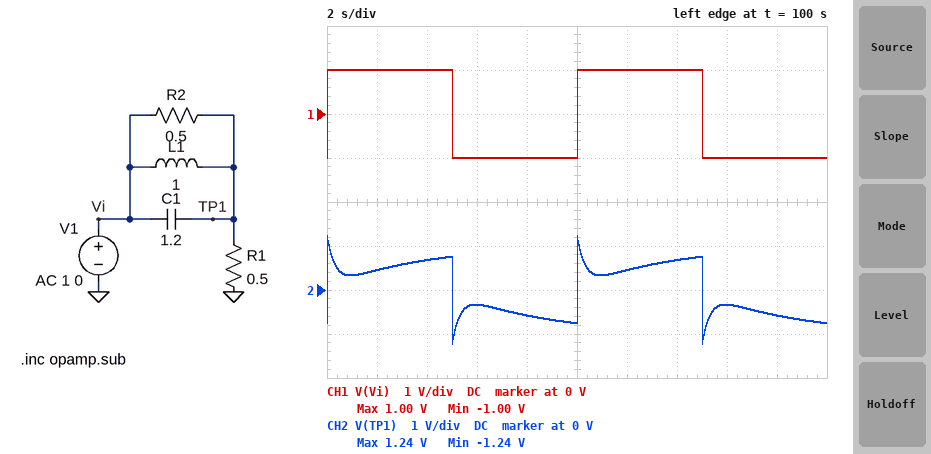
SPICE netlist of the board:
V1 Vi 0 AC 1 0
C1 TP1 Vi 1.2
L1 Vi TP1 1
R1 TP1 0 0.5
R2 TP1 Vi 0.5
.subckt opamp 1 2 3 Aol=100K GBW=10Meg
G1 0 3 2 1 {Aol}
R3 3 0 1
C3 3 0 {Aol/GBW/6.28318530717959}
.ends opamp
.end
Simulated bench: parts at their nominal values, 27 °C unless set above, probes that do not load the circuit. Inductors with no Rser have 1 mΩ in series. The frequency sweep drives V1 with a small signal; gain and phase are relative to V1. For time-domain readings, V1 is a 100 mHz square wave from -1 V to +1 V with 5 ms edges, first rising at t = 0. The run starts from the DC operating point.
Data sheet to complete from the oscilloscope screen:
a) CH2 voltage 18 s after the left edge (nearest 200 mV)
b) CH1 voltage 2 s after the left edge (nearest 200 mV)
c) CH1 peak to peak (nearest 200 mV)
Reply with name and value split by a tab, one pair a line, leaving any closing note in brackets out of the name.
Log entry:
CH2 voltage 18 s after the left edge	-600 mV
CH1 voltage 2 s after the left edge	1.0 V
CH1 peak to peak	2.0 V
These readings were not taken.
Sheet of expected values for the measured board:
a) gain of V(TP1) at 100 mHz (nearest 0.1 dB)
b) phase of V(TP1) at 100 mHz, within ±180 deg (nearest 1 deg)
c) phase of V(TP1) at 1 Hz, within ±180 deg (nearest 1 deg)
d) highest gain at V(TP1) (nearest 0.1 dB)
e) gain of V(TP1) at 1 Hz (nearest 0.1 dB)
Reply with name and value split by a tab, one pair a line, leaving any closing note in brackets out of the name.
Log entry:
gain of V(TP1) at 100 mHz	-5.5 dB
phase of V(TP1) at 100 mHz, within ±180 deg	-11 deg
phase of V(TP1) at 1 Hz, within ±180 deg	13 deg
highest gain at V(TP1)	0 dB
gain of V(TP1) at 1 Hz	-0.8 dB
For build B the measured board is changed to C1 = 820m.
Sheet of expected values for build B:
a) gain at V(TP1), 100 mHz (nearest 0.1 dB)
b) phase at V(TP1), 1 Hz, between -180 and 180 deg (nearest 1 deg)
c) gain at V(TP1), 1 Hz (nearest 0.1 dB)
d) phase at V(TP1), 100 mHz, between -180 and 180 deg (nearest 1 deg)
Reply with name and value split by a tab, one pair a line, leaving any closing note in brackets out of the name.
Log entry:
gain at V(TP1), 100 mHz	-5.2 dB
phase at V(TP1), 1 Hz, between -180 and 180 deg	17 deg
gain at V(TP1), 1 Hz	-1.5 dB
phase at V(TP1), 100 mHz, between -180 and 180 deg	-13 deg
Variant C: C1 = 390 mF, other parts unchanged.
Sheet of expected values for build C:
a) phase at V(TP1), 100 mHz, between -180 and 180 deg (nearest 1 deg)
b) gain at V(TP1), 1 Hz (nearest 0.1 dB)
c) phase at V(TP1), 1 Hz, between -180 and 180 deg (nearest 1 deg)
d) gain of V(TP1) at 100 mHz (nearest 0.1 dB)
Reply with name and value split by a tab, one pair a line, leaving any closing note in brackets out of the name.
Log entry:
phase at V(TP1), 100 mHz, between -180 and 180 deg	-15 deg
gain at V(TP1), 1 Hz	-3.6 dB
phase at V(TP1), 1 Hz, between -180 and 180 deg	19 deg
gain of V(TP1) at 100 mHz	-4.9 dB
